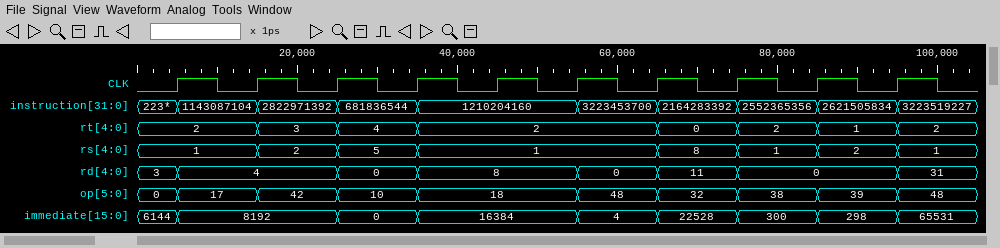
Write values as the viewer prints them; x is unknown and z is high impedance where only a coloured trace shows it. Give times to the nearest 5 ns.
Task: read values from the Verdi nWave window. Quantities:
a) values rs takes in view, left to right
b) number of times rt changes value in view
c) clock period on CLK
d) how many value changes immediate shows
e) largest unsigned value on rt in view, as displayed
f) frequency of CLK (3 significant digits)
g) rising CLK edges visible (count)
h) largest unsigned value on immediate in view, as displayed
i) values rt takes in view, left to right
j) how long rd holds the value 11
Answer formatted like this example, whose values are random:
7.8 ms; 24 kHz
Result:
1, 2, 5, 1, 8, 1, 2, 1; 7; 10 ns; 8; 4; 100 MHz; 10; 65531; 2, 3, 4, 2, 0, 2, 1, 2; 10 ns
